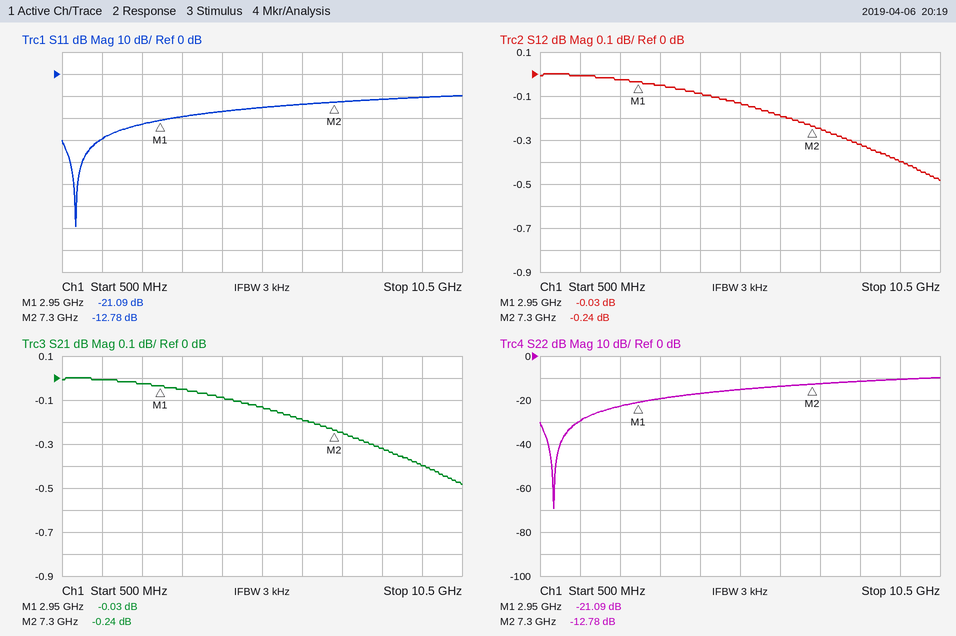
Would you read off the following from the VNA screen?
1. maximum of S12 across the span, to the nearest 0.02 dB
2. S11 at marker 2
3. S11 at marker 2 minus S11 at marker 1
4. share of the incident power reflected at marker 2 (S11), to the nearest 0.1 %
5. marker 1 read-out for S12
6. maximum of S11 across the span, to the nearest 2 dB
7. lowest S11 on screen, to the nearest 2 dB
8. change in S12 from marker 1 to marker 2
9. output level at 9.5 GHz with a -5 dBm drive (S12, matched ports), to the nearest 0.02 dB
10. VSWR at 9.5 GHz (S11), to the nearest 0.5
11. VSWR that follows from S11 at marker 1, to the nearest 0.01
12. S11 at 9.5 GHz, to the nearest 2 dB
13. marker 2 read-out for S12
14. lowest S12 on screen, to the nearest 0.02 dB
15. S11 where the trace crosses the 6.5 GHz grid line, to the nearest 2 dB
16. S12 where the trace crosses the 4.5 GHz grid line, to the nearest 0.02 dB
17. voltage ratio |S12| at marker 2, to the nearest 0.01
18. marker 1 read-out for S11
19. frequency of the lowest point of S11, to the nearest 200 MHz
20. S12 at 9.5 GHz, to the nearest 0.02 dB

0.00 dB
-12.78 dB
8.31 dB
5.3 %
-0.03 dB
-10 dB
-70 dB
-0.21 dB
-5.40 dBm
2.0
1.19
-10 dB
-0.24 dB
-0.48 dB
-14 dB
-0.08 dB
0.97
-21.09 dB
800 MHz
-0.40 dB
